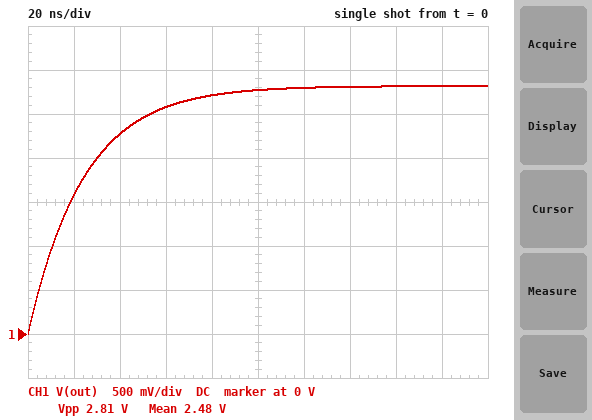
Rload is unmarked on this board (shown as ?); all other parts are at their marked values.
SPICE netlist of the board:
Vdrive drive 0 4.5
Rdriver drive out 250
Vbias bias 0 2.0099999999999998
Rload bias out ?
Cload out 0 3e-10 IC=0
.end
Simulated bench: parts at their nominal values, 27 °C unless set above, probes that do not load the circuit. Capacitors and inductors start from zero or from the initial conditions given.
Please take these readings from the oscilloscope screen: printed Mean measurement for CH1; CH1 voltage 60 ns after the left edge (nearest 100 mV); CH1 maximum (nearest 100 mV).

2.48 V
2.6 V
2.8 V
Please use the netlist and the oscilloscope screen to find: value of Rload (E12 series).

120 Ω
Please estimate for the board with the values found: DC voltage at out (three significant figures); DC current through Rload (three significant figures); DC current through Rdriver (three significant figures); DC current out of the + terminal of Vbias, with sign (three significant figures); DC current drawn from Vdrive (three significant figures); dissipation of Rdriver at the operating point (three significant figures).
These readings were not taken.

2.82 V
6.73 mA
6.73 mA
-6.73 mA
6.73 mA
11.3 mW
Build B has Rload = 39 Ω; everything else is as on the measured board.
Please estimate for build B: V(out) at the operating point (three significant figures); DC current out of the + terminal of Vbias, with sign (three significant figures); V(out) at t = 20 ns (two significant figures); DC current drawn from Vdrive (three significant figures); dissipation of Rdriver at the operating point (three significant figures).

2.35 V
-8.62 mA
2.0 V
8.62 mA
18.6 mW
